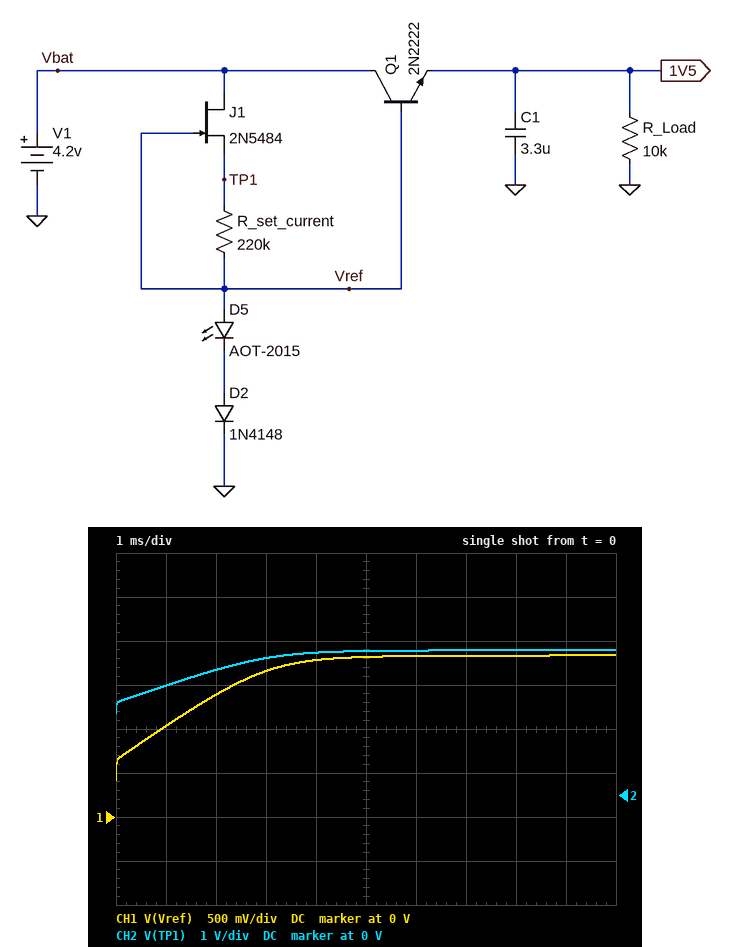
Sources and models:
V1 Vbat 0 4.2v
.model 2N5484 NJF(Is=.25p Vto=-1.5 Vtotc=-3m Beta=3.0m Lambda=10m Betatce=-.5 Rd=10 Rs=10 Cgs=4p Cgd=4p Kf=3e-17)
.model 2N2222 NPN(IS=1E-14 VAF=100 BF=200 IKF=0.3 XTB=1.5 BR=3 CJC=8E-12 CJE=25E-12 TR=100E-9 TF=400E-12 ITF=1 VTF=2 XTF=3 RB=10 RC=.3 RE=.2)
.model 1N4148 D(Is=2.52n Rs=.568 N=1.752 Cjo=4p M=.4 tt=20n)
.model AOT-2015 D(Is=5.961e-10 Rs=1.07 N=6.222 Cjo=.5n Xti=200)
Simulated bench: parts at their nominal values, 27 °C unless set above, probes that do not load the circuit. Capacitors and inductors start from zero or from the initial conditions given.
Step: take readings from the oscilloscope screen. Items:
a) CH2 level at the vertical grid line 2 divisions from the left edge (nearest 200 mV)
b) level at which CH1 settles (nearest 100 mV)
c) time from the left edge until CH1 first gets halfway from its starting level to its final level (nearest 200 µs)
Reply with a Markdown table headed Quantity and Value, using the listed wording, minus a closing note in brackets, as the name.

| Quantity | Value |
|---|---|
| CH2 level at the vertical grid line 2 divisions from the left edge | 2.8 V |
| level at which CH1 settles | 1.8 V |
| time from the left edge until CH1 first gets halfway from its starting level to its final level | 1.4 ms |
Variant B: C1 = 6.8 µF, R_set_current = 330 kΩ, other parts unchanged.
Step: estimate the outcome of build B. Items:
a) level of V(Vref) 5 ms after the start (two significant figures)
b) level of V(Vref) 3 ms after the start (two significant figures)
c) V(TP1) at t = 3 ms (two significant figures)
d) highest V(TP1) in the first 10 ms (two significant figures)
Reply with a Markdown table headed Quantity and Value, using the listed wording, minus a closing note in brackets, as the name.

| Quantity | Value |
|---|---|
| level of V(Vref) 5 ms after the start | 1.3 V |
| level of V(Vref) 3 ms after the start | 1.0 V |
| V(TP1) at t = 3 ms | 2.5 V |
| highest V(TP1) in the first 10 ms | 3.1 V |
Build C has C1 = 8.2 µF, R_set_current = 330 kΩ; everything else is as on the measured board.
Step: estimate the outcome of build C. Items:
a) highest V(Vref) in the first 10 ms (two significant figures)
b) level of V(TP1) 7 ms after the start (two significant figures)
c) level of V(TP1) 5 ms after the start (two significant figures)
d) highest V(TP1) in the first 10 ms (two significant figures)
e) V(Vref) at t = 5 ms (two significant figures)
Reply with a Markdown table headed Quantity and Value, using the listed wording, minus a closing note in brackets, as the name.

| Quantity | Value |
|---|---|
| highest V(Vref) in the first 10 ms | 1.6 V |
| level of V(TP1) 7 ms after the start | 2.8 V |
| level of V(TP1) 5 ms after the start | 2.6 V |
| highest V(TP1) in the first 10 ms | 3.0 V |
| V(Vref) at t = 5 ms | 1.2 V |
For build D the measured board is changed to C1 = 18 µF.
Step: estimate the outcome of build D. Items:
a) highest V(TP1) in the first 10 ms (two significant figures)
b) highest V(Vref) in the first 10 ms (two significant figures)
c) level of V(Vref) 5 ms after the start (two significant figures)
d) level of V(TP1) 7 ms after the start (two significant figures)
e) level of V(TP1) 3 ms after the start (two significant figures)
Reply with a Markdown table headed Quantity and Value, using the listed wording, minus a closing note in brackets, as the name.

| Quantity | Value |
|---|---|
| highest V(TP1) in the first 10 ms | 2.8 V |
| highest V(Vref) in the first 10 ms | 1.4 V |
| level of V(Vref) 5 ms after the start | 1.0 V |
| level of V(TP1) 7 ms after the start | 2.6 V |
| level of V(TP1) 3 ms after the start | 2.3 V |
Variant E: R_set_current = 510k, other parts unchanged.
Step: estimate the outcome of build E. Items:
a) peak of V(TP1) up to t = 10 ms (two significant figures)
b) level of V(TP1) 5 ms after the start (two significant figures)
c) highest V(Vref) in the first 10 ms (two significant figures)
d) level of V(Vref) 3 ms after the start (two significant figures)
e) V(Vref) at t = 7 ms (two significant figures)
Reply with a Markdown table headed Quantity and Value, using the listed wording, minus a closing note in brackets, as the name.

| Quantity | Value |
|---|---|
| peak of V(TP1) up to t = 10 ms | 3.1 V |
| level of V(TP1) 5 ms after the start | 2.8 V |
| highest V(Vref) in the first 10 ms | 1.6 V |
| level of V(Vref) 3 ms after the start | 1.1 V |
| V(Vref) at t = 7 ms | 1.5 V |
